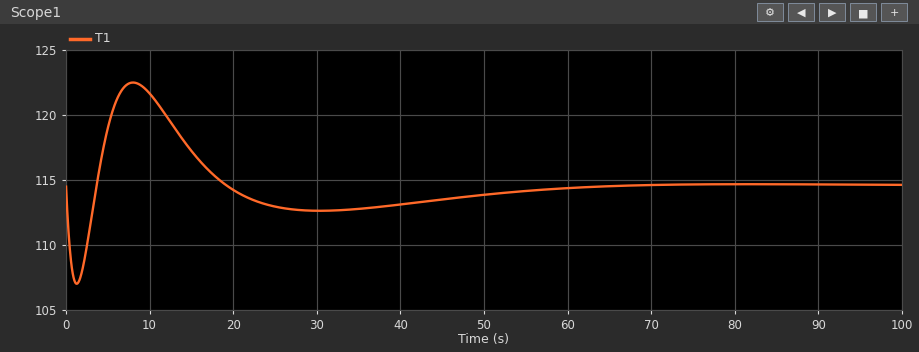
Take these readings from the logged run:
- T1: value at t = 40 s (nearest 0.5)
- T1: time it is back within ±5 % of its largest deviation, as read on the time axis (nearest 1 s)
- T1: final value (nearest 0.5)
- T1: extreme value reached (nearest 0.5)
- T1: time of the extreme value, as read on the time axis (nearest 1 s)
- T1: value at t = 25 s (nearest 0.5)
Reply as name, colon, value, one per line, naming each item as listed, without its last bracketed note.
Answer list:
T1: value at t = 40 s: 113.0
T1: time it is back within ±5 % of its largest deviation, as read on the time axis: 56 s
T1: final value: 114.5
T1: extreme value reached: 122.5
T1: time of the extreme value, as read on the time axis: 8 s
T1: value at t = 25 s: 113.0
